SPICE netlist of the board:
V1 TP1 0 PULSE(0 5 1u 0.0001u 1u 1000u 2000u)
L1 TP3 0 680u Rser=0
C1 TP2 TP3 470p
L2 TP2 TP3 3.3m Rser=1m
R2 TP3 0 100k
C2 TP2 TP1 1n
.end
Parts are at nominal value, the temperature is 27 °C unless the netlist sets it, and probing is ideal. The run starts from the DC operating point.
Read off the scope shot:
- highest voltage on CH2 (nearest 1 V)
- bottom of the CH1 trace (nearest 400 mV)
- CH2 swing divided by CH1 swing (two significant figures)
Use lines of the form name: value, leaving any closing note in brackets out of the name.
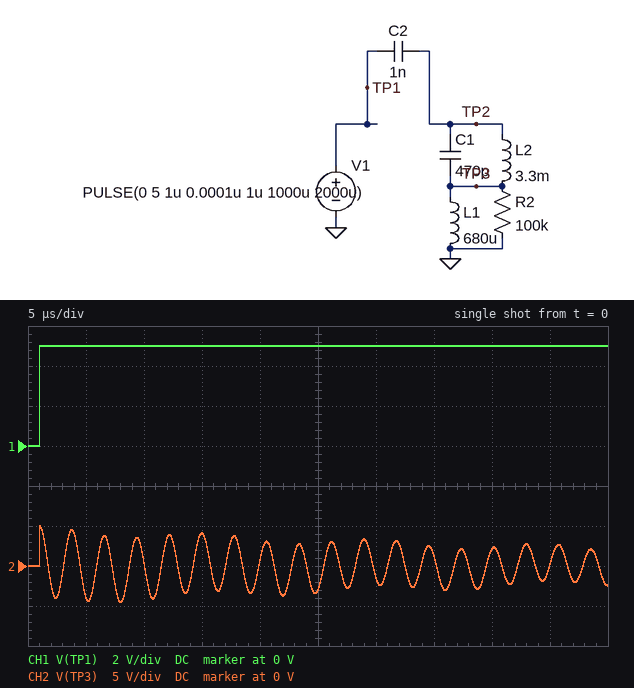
highest voltage on CH2: 5 V
bottom of the CH1 trace: 0 V
CH2 swing divided by CH1 swing: 1.9
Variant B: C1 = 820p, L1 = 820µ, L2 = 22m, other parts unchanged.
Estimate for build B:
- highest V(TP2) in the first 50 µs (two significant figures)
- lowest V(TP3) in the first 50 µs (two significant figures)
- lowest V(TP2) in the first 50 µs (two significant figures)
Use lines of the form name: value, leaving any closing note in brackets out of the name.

highest V(TP2) in the first 50 µs: 5.0 V
lowest V(TP3) in the first 50 µs: -4.8 V
lowest V(TP2) in the first 50 µs: -4.5 V
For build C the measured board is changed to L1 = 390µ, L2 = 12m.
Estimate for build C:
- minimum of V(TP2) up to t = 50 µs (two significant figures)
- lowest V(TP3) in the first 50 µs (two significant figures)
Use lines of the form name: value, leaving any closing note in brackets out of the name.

minimum of V(TP2) up to t = 50 µs: -4.6 V
lowest V(TP3) in the first 50 µs: -4.8 V
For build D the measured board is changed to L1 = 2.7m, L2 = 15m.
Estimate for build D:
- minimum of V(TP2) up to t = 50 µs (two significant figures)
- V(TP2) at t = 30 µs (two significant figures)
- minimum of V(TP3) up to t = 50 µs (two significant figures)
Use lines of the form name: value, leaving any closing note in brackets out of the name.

minimum of V(TP2) up to t = 50 µs: -4.6 V
V(TP2) at t = 30 µs: 3.8 V
minimum of V(TP3) up to t = 50 µs: -4.1 V
